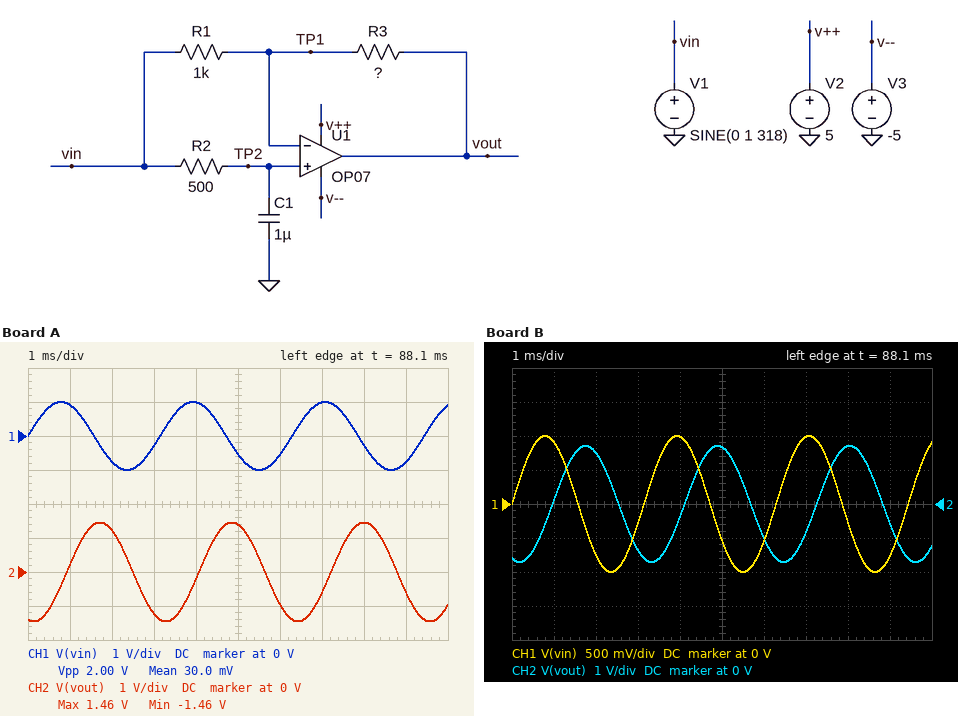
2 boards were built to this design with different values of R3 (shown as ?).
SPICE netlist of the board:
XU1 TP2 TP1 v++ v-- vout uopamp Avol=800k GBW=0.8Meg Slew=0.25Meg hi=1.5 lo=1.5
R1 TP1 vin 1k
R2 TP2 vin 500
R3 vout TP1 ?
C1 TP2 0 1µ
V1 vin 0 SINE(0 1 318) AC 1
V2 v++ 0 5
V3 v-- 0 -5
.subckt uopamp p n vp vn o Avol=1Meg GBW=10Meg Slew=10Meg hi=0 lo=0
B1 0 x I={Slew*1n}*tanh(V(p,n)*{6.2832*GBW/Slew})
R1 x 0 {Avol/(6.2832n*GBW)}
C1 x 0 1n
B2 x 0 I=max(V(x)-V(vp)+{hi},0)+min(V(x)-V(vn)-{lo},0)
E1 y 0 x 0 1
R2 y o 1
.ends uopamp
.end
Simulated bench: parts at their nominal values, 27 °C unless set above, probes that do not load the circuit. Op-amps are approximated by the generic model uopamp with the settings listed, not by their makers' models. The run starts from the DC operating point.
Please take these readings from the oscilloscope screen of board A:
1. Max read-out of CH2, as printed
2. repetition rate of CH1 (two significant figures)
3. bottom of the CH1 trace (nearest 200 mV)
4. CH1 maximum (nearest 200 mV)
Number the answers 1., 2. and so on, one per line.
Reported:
1. 1.46 V
2. 320 Hz
3. -1.0 V
4. 1.0 V
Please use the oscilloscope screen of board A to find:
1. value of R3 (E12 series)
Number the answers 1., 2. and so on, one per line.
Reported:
1. 1.8 kΩ
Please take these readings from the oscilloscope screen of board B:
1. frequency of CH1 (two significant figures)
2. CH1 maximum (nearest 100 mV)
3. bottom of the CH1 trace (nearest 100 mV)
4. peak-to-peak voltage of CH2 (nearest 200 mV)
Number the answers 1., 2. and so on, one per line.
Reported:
1. 320 Hz
2. 1.0 V
3. -1.0 V
4. 3.4 V
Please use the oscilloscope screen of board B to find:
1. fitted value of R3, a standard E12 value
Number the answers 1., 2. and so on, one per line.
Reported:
1. 2.2 kΩ
